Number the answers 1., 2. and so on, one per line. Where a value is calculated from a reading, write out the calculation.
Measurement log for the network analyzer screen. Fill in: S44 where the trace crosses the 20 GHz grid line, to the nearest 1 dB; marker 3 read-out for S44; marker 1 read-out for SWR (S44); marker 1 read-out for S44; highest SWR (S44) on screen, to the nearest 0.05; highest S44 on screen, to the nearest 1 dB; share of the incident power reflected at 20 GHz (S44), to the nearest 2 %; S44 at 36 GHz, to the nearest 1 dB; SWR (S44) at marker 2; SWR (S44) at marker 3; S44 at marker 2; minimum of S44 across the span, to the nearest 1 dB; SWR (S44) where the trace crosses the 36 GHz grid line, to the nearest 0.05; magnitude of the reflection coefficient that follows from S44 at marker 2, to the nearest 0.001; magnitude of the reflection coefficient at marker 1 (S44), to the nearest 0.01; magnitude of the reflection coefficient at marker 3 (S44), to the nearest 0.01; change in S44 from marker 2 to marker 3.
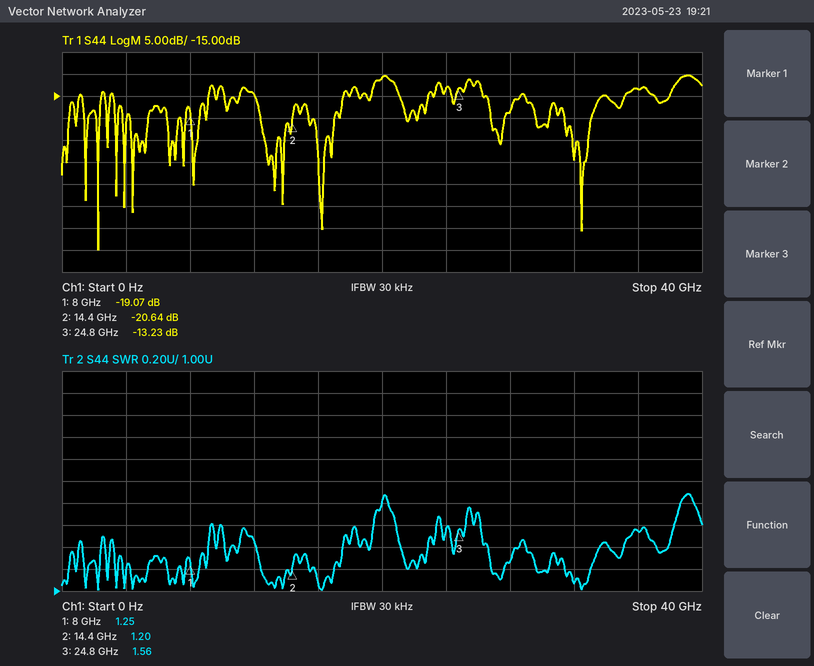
1. -11 dB
2. -13.23 dB
3. 1.25
4. -19.07 dB
5. 1.90
6. -10 dB
7. 10^(-11/10) ≈ 8 %
8. -13 dB
9. 1.20
10. 1.56
11. -20.64 dB
12. -50 dB
13. 1.55
14. 10^(-20.64/20) ≈ 0.093
15. 10^(-19.07/20) ≈ 0.11
16. 10^(-13.23/20) ≈ 0.22
17. -13.23 − (-20.64) = 7.41 dB
